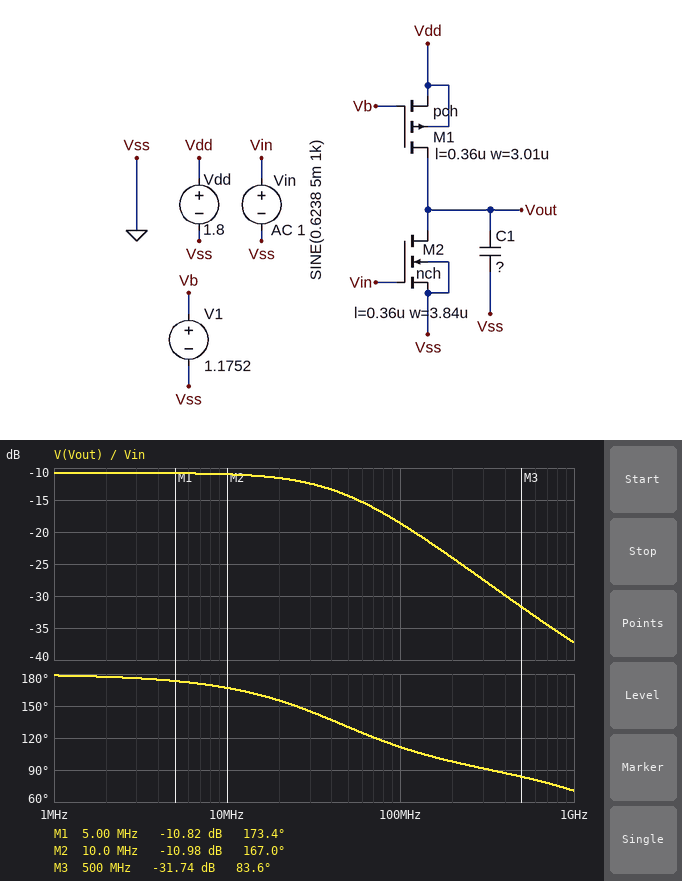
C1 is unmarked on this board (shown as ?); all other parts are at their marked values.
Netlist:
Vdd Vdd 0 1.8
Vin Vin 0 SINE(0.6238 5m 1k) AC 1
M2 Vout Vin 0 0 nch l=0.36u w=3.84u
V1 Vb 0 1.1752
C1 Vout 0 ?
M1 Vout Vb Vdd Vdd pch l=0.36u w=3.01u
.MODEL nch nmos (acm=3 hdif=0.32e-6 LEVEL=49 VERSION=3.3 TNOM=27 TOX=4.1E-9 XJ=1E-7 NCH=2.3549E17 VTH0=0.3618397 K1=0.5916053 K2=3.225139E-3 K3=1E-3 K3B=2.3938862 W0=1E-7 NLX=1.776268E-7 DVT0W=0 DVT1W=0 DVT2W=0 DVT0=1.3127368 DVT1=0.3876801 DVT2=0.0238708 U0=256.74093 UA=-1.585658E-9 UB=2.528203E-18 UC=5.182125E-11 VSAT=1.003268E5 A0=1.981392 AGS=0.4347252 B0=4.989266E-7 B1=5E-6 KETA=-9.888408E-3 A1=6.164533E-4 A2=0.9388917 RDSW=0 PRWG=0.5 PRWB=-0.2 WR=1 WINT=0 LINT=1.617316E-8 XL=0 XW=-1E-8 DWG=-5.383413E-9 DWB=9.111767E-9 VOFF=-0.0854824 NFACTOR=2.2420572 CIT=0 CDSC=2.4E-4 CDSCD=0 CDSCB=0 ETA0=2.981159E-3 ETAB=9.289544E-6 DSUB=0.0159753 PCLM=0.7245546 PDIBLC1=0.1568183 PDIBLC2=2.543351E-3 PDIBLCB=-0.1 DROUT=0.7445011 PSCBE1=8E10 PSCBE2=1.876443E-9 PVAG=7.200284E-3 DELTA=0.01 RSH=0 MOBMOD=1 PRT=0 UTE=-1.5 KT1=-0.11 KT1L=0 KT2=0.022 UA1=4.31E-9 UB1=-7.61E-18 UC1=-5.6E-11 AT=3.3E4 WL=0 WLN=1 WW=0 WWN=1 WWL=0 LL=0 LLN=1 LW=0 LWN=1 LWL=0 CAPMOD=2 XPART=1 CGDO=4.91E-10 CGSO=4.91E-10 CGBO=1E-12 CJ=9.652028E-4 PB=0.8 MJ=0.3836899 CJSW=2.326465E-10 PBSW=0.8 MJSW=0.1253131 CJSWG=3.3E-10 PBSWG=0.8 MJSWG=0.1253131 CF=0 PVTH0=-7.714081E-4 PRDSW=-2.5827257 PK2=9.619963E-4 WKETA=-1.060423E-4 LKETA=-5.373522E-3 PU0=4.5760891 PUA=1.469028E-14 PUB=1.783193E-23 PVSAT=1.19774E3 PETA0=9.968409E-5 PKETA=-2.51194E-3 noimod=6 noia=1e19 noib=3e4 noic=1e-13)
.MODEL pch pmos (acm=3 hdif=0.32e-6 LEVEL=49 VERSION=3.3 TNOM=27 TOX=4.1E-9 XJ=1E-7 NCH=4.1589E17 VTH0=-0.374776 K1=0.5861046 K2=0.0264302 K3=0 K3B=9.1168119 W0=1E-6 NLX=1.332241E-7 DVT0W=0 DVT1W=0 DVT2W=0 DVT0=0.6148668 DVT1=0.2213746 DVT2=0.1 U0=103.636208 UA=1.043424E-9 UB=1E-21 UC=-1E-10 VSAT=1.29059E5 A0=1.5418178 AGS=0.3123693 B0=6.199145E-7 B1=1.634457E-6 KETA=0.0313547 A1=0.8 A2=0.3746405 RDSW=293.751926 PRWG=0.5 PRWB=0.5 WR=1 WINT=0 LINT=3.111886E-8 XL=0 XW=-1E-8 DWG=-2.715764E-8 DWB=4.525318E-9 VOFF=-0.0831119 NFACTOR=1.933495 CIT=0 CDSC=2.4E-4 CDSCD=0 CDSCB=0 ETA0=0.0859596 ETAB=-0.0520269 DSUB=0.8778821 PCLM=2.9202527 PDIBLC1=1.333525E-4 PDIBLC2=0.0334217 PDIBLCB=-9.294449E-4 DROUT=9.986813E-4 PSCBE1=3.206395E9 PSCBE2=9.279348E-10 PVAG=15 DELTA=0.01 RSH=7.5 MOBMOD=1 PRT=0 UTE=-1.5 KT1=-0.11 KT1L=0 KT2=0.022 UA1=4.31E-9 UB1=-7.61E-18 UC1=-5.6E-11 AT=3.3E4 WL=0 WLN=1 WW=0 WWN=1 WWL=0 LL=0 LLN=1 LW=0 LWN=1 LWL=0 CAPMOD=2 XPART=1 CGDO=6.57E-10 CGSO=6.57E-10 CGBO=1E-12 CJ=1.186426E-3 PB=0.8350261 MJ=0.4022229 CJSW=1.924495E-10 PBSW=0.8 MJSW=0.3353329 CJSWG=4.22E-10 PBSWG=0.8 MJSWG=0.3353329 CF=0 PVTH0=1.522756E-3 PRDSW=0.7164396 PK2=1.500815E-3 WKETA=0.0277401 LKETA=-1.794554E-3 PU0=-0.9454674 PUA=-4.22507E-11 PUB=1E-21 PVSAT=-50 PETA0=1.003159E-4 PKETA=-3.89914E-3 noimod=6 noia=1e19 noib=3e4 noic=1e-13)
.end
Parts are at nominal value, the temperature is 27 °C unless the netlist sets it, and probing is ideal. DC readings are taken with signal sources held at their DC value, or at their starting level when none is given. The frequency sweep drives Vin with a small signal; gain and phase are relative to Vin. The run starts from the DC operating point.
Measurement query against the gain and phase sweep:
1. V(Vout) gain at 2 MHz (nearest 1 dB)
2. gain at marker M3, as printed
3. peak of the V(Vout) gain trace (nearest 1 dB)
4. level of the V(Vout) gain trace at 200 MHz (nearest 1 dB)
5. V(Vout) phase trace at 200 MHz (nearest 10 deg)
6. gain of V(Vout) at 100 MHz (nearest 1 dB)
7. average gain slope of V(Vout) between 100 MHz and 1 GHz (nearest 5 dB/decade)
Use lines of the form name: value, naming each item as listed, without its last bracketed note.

V(Vout) gain at 2 MHz: -11 dB
gain at marker M3, as printed: -31.74 dB
peak of the V(Vout) gain trace: -11 dB
level of the V(Vout) gain trace at 200 MHz: -24 dB
V(Vout) phase trace at 200 MHz: 100 deg
gain of V(Vout) at 100 MHz: -19 dB
average gain slope of V(Vout) between 100 MHz and 1 GHz: -20 dB/decade
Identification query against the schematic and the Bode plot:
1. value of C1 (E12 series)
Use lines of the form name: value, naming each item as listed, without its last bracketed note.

value of C1: 1.2 pF
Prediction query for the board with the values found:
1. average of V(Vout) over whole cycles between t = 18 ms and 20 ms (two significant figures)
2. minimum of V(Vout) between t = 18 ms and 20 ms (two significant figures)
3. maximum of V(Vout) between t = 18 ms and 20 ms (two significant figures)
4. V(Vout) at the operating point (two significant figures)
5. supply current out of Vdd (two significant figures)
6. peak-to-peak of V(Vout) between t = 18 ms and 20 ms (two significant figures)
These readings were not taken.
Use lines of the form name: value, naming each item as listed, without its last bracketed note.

average of V(Vout) over whole cycles between t = 18 ms and 20 ms: 29 mV
minimum of V(Vout) between t = 18 ms and 20 ms: 28 mV
maximum of V(Vout) between t = 18 ms and 20 ms: 31 mV
V(Vout) at the operating point: 29 mV
supply current out of Vdd: 11 µA
peak-to-peak of V(Vout) between t = 18 ms and 20 ms: 2.9 mV
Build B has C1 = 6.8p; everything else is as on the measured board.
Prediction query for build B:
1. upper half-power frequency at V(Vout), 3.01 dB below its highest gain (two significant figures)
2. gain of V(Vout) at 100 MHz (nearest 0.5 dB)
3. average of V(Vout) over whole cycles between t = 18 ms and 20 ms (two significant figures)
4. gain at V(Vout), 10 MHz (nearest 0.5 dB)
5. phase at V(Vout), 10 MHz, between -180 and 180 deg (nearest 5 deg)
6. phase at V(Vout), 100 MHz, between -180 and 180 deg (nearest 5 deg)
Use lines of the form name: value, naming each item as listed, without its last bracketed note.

upper half-power frequency at V(Vout), 3.01 dB below its highest gain: 7.9 MHz
gain of V(Vout) at 100 MHz: -33.0 dB
average of V(Vout) over whole cycles between t = 18 ms and 20 ms: 29 mV
gain at V(Vout), 10 MHz: -15.0 dB
phase at V(Vout), 10 MHz, between -180 and 180 deg: 130 deg
phase at V(Vout), 100 MHz, between -180 and 180 deg: 90 deg
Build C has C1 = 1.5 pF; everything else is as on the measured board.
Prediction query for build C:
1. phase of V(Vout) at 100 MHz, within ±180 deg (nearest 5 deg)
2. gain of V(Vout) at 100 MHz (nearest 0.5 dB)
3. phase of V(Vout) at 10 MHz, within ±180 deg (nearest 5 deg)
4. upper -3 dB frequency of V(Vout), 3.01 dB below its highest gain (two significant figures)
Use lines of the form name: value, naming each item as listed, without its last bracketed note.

phase of V(Vout) at 100 MHz, within ±180 deg: 105 deg
gain of V(Vout) at 100 MHz: -20.5 dB
phase of V(Vout) at 10 MHz, within ±180 deg: 165 deg
upper -3 dB frequency of V(Vout), 3.01 dB below its highest gain: 35 MHz
